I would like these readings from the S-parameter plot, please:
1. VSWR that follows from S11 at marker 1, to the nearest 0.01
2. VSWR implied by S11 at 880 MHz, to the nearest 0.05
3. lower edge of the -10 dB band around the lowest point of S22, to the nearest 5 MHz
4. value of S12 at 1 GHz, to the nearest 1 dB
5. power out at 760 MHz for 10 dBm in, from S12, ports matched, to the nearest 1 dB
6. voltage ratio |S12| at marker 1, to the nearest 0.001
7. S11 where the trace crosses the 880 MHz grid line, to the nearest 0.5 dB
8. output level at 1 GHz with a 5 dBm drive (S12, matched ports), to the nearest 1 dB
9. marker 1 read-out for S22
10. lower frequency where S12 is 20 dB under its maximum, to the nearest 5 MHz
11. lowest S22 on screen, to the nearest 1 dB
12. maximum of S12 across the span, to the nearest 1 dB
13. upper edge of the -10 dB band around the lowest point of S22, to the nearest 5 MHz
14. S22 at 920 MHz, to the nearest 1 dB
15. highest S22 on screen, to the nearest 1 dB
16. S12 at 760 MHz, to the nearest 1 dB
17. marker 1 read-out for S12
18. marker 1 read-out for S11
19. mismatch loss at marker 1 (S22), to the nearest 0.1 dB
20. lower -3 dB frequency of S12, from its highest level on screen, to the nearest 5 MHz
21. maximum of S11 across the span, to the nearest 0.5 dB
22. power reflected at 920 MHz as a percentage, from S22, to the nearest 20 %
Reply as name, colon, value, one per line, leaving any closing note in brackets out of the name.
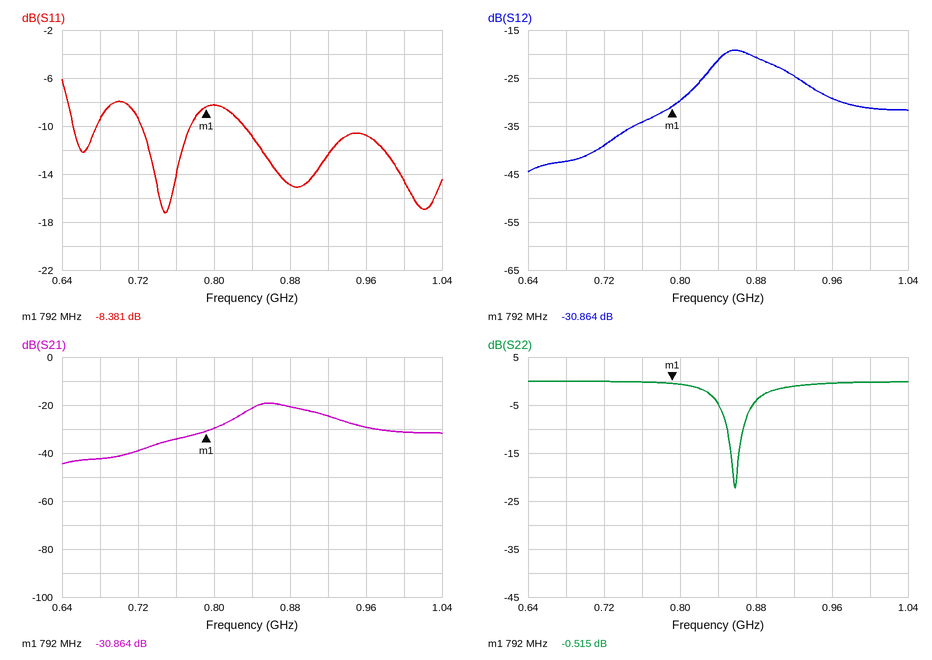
VSWR that follows from S11 at marker 1, to the nearest 0.01: 2.23
VSWR implied by S11 at 880 MHz, to the nearest 0.05: 1.45
lower edge of the -10 dB band around the lowest point of S22, to the nearest 5 MHz: 850 MHz
value of S12 at 1 GHz, to the nearest 1 dB: -31 dB
power out at 760 MHz for 10 dBm in, from S12, ports matched, to the nearest 1 dB: -24 dBm
voltage ratio |S12| at marker 1, to the nearest 0.001: 0.029
S11 where the trace crosses the 880 MHz grid line, to the nearest 0.5 dB: -15.0 dB
output level at 1 GHz with a 5 dBm drive (S12, matched ports), to the nearest 1 dB: -26 dBm
marker 1 read-out for S22: -0.515 dB
lower frequency where S12 is 20 dB under its maximum, to the nearest 5 MHz: 720 MHz
lowest S22 on screen, to the nearest 1 dB: -22 dB
maximum of S12 across the span, to the nearest 1 dB: -19 dB
upper edge of the -10 dB band around the lowest point of S22, to the nearest 5 MHz: 865 MHz
S22 at 920 MHz, to the nearest 1 dB: -1 dB
highest S22 on screen, to the nearest 1 dB: 0 dB
S12 at 760 MHz, to the nearest 1 dB: -34 dB
marker 1 read-out for S12: -30.864 dB
marker 1 read-out for S11: -8.381 dB
mismatch loss at marker 1 (S22), to the nearest 0.1 dB: 9.5 dB
lower -3 dB frequency of S12, from its highest level on screen, to the nearest 5 MHz: 835 MHz
maximum of S11 across the span, to the nearest 0.5 dB: -6.0 dB
power reflected at 920 MHz as a percentage, from S22, to the nearest 20 %: 80 %
